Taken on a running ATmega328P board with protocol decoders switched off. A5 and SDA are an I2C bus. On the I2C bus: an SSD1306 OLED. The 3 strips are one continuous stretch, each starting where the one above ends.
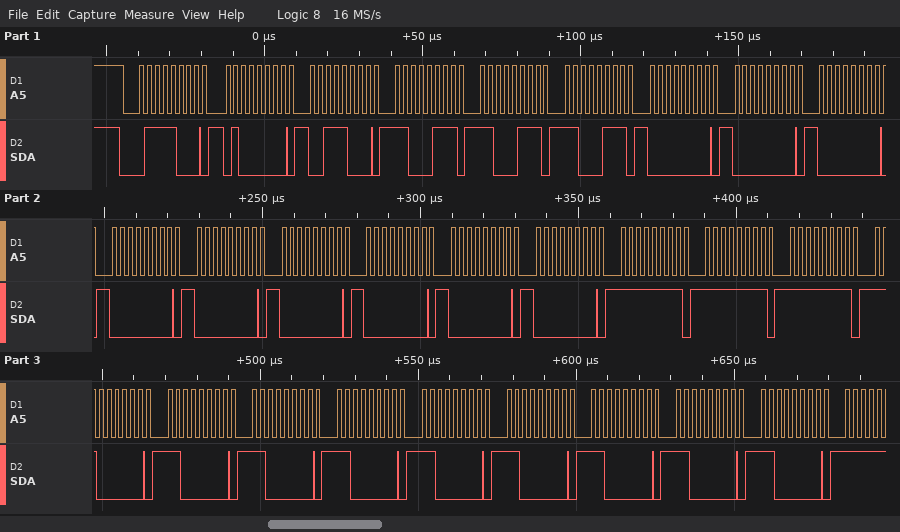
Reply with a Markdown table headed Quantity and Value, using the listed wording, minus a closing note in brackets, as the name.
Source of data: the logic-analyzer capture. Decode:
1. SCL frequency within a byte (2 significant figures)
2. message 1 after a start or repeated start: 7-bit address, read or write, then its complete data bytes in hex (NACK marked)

| Quantity | Value |
|---|---|
| SCL frequency within a byte | 400 kHz |
| message 1 after a start or repeated start: 7-bit address, read or write, then its complete data bytes in hex | 0x3C write: 40 38 C7 C7 C7 00 00 00 00 00 00 00 00 00 FF FF FF C0 C0 C0 C0 C0 C0 C0 C0 C0 |
